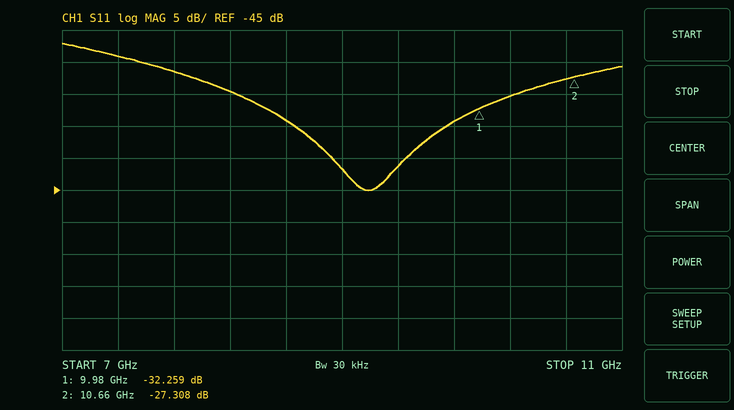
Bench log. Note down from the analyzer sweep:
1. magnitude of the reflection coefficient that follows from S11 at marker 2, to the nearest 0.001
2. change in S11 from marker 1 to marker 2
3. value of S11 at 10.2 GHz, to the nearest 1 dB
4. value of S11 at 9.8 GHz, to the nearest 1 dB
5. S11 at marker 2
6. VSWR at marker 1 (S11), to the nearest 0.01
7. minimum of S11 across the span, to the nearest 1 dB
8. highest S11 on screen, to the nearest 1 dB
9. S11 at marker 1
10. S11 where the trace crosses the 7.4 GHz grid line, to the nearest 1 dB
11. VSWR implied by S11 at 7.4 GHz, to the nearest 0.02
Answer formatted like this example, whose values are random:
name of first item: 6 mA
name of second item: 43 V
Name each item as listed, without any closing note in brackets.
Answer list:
magnitude of the reflection coefficient that follows from S11 at marker 2, to the nearest 0.001: 0.043
change in S11 from marker 1 to marker 2: 4.951 dB
value of S11 at 10.2 GHz, to the nearest 1 dB: -30 dB
value of S11 at 9.8 GHz, to the nearest 1 dB: -34 dB
S11 at marker 2: -27.308 dB
VSWR at marker 1 (S11), to the nearest 0.01: 1.05
minimum of S11 across the span, to the nearest 1 dB: -45 dB
highest S11 on screen, to the nearest 1 dB: -22 dB
S11 at marker 1: -32.259 dB
S11 where the trace crosses the 7.4 GHz grid line, to the nearest 1 dB: -24 dB
VSWR implied by S11 at 7.4 GHz, to the nearest 0.02: 1.14
